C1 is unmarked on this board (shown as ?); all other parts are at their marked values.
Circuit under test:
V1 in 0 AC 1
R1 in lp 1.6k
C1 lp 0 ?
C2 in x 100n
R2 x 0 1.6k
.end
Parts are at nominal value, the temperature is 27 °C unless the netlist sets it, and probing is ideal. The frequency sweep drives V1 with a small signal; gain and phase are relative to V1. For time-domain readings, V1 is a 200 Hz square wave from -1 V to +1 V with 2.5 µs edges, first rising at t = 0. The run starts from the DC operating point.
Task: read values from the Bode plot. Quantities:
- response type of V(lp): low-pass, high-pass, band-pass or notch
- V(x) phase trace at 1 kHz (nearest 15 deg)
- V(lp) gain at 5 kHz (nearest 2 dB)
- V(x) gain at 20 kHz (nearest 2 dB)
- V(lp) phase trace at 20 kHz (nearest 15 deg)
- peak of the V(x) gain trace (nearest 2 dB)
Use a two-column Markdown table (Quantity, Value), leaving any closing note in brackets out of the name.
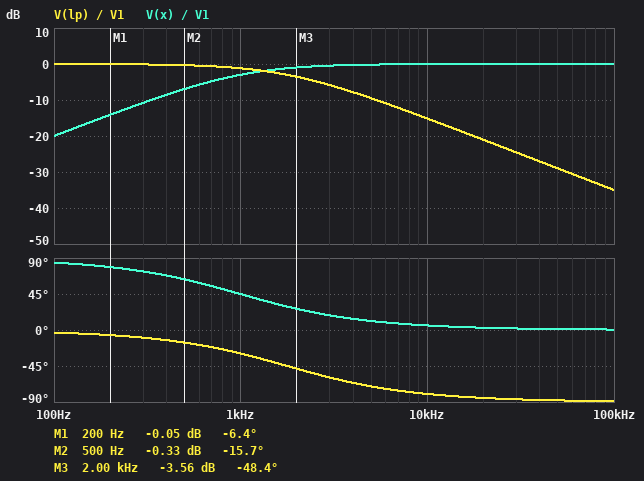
| Quantity | Value |
|---|---|
| response type of V(lp): low-pass, high-pass, band-pass or notch | low-pass |
| V(x) phase trace at 1 kHz | 45 deg |
| V(lp) gain at 5 kHz | -10 dB |
| V(x) gain at 20 kHz | 0 dB |
| V(lp) phase trace at 20 kHz | -90 deg |
| peak of the V(x) gain trace | 0 dB |
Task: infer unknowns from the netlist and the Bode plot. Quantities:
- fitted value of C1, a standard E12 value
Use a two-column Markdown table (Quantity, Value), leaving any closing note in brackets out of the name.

| Quantity | Value |
|---|---|
| fitted value of C1, a standard E12 value | 56 nF |
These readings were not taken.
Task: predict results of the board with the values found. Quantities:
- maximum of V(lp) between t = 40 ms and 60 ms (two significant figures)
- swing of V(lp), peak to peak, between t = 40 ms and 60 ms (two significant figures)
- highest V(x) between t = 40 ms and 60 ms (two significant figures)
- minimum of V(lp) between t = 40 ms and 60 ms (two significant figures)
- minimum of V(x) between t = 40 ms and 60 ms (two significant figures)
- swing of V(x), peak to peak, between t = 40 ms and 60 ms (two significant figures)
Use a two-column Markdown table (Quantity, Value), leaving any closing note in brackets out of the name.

| Quantity | Value |
|---|---|
| maximum of V(lp) between t = 40 ms and 60 ms | 1.0 V |
| swing of V(lp), peak to peak, between t = 40 ms and 60 ms | 2.0 V |
| highest V(x) between t = 40 ms and 60 ms | 2.0 V |
| minimum of V(lp) between t = 40 ms and 60 ms | -1.0 V |
| minimum of V(x) between t = 40 ms and 60 ms | -2.0 V |
| swing of V(x), peak to peak, between t = 40 ms and 60 ms | 4.0 V |
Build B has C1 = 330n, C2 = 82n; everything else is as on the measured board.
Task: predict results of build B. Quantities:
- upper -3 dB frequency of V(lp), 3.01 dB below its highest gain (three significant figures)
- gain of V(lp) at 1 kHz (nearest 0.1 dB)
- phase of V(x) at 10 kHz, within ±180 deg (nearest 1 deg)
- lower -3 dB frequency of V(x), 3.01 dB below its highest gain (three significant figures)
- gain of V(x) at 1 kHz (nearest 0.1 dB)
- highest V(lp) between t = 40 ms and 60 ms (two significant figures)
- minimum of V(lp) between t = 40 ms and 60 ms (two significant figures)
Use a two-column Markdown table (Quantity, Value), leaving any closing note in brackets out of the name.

| Quantity | Value |
|---|---|
| upper -3 dB frequency of V(lp), 3.01 dB below its highest gain | 301 Hz |
| gain of V(lp) at 1 kHz | -10.8 dB |
| phase of V(x) at 10 kHz, within ±180 deg | 7 deg |
| lower -3 dB frequency of V(x), 3.01 dB below its highest gain | 1.21 kHz |
| gain of V(x) at 1 kHz | -3.9 dB |
| highest V(lp) between t = 40 ms and 60 ms | 980 mV |
| minimum of V(lp) between t = 40 ms and 60 ms | -980 mV |
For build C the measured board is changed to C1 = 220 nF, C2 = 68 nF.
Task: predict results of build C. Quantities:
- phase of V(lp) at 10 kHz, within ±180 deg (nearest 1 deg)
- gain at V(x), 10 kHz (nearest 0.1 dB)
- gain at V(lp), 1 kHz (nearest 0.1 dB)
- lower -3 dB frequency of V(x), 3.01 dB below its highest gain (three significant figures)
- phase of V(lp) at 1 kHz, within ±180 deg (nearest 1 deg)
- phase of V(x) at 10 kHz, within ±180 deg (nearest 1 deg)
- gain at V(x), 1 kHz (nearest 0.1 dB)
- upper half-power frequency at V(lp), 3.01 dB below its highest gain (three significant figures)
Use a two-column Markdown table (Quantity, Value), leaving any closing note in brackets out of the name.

| Quantity | Value |
|---|---|
| phase of V(lp) at 10 kHz, within ±180 deg | -87 deg |
| gain at V(x), 10 kHz | -0.1 dB |
| gain at V(lp), 1 kHz | -7.7 dB |
| lower -3 dB frequency of V(x), 3.01 dB below its highest gain | 1.46 kHz |
| phase of V(lp) at 1 kHz, within ±180 deg | -66 deg |
| phase of V(x) at 10 kHz, within ±180 deg | 8 deg |
| gain at V(x), 1 kHz | -5.0 dB |
| upper half-power frequency at V(lp), 3.01 dB below its highest gain | 452 Hz |
